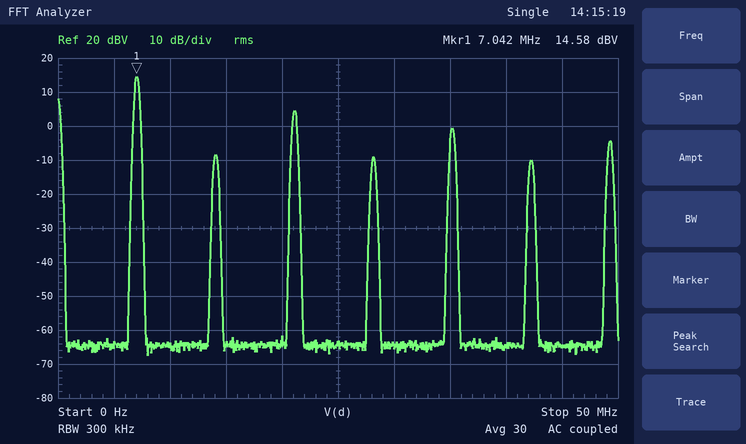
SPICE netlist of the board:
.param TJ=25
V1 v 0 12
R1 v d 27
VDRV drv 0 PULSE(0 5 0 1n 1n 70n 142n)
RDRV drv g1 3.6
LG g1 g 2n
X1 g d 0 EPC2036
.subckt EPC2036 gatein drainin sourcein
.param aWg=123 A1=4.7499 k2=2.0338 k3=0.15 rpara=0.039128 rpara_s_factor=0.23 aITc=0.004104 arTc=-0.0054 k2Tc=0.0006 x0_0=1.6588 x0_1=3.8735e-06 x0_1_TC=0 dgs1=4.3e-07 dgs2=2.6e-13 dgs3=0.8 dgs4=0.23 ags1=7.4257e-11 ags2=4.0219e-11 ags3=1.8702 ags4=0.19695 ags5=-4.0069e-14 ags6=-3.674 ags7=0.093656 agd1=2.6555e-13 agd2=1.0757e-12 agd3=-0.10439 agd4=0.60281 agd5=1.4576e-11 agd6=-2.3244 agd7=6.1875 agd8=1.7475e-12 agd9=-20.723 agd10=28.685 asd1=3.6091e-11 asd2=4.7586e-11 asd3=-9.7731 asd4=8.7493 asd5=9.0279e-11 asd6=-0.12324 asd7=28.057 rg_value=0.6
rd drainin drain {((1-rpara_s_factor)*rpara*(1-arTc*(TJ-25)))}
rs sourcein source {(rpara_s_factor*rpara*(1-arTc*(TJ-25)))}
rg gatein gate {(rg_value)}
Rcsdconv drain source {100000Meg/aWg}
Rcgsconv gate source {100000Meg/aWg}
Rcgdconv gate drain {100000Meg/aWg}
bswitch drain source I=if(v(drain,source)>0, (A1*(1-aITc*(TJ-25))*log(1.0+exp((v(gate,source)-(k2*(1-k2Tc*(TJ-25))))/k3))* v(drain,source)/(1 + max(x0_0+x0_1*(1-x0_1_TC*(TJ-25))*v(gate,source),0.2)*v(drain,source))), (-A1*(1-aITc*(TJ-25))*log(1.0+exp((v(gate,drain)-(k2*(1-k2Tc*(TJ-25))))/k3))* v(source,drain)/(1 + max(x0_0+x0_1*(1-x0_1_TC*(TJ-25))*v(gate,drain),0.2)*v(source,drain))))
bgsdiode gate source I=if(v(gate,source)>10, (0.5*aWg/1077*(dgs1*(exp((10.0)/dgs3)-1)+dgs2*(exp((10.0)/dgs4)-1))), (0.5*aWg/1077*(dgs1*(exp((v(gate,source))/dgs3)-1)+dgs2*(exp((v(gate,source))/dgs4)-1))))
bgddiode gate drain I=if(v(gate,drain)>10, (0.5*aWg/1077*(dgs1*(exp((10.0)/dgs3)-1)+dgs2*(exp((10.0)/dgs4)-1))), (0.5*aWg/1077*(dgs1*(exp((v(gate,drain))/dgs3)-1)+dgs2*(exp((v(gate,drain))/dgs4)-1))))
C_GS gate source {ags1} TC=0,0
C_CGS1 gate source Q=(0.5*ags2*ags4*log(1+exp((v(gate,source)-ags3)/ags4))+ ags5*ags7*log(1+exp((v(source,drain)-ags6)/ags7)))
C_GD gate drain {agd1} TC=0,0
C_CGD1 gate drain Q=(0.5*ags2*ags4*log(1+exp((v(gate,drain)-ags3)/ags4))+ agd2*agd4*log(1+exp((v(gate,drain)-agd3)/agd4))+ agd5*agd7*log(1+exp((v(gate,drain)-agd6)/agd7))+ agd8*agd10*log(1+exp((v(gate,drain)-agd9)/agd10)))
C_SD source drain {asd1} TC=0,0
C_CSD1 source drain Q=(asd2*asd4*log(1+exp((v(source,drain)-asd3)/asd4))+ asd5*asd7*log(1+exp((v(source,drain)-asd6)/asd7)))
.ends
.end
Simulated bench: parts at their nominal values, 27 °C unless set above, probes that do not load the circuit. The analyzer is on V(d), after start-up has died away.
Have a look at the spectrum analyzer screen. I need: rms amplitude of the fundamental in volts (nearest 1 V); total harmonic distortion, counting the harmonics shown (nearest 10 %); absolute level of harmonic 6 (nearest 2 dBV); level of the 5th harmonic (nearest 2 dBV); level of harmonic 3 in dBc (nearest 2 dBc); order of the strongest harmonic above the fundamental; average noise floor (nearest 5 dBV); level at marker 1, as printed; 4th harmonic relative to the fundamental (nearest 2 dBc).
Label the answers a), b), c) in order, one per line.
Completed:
a) 5 V
b) 40 %
c) -10 dBV
d) 0 dBV
e) -10 dBc
f) 3
g) -65 dBV
h) 14.58 dBV
i) -24 dBc
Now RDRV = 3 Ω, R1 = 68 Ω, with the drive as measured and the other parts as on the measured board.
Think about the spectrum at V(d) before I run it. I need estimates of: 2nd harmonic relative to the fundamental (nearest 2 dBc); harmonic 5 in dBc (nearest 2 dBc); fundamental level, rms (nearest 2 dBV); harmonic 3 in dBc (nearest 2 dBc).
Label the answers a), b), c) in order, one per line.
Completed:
a) -16 dBc
b) -18 dBc
c) 14 dBV
d) -12 dBc
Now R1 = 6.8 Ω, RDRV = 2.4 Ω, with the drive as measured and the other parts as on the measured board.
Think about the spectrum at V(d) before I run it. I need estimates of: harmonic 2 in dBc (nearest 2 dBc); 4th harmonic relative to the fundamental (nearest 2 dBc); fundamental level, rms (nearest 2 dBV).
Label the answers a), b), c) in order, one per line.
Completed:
a) -34 dBc
b) -34 dBc
c) 14 dBV
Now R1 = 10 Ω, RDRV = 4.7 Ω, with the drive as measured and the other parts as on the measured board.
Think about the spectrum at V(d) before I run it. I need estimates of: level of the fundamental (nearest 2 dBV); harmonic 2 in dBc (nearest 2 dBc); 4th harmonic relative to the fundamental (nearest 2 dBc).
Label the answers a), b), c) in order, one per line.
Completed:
a) 14 dBV
b) -30 dBc
c) -30 dBc
